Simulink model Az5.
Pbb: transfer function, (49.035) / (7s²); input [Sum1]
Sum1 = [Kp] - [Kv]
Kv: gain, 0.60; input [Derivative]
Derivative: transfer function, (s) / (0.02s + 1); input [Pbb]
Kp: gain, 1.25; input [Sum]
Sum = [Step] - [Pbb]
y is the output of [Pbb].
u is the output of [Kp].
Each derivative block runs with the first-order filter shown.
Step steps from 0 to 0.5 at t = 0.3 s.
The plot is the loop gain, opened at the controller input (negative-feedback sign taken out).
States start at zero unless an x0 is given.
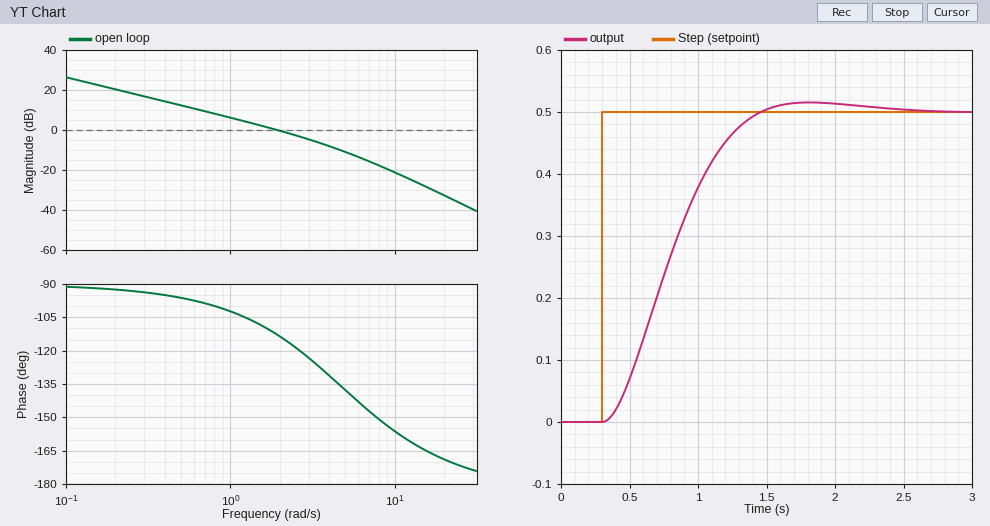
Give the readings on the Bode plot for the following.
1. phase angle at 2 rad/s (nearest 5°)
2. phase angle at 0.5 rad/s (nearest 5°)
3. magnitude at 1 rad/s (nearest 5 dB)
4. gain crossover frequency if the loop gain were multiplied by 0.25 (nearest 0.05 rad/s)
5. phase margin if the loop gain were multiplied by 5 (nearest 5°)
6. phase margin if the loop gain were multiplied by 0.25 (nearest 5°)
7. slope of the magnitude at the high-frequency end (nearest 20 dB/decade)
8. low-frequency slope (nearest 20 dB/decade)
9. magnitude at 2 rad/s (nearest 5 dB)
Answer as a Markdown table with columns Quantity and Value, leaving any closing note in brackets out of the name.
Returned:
| Quantity | Value |
|---|---|
| phase angle at 2 rad/s | -115° |
| phase angle at 0.5 rad/s | -95° |
| magnitude at 1 rad/s | 5 dB |
| gain crossover frequency if the loop gain were multiplied by 0.25 | 0.50 rad/s |
| phase margin if the loop gain were multiplied by 5 | 35° |
| phase margin if the loop gain were multiplied by 0.25 | 85° |
| slope of the magnitude at the high-frequency end | -40 dB/decade |
| low-frequency slope | -20 dB/decade |
| magnitude at 2 rad/s | 0 dB |
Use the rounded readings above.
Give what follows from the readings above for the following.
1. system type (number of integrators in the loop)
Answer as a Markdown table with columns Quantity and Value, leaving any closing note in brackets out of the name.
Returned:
| Quantity | Value |
|---|---|
| system type | 1 |
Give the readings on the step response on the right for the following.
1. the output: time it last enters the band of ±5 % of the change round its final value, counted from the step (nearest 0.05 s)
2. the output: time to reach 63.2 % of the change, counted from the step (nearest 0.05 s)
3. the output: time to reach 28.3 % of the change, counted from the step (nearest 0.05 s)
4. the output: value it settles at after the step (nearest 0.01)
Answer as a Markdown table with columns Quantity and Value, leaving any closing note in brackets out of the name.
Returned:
| Quantity | Value |
|---|---|
| the output: time it last enters the band of ±5 % of the change round its final value, counted from the step | 1.00 s |
| the output: time to reach 63.2 % of the change, counted from the step | 0.60 s |
| the output: time to reach 28.3 % of the change, counted from the step | 0.30 s |
| the output: value it settles at after the step | 0.50 |
